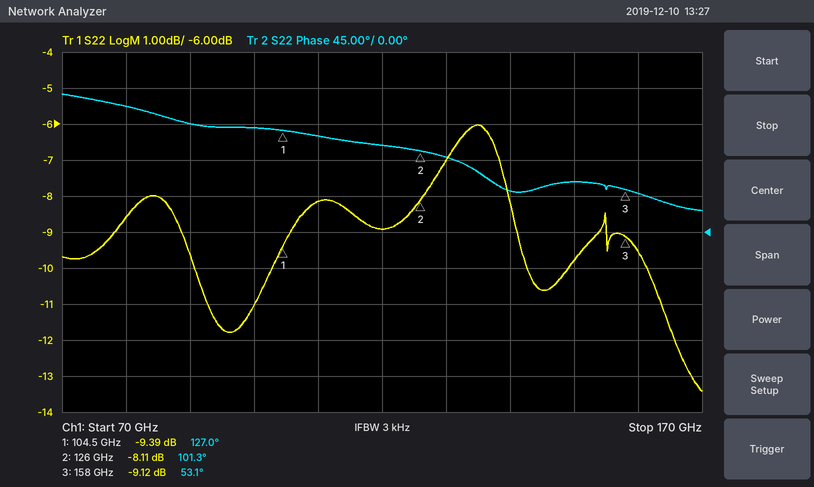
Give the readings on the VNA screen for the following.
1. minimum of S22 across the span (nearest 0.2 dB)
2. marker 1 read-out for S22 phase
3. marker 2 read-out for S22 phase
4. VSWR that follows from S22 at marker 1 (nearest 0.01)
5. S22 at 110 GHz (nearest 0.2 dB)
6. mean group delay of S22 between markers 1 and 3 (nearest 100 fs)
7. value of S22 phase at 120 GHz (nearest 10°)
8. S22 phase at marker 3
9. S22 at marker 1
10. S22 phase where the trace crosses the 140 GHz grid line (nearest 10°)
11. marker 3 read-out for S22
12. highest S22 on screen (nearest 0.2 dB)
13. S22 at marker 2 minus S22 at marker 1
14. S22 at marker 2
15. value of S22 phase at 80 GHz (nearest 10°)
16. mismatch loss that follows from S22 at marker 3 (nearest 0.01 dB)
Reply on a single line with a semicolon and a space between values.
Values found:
-13.4 dB; 127.0°; 101.3°; 2.03; -8.2 dB; 3.8 ps; 110°; 53.1°; -9.39 dB; 50°; -9.12 dB; -6.0 dB; 1.28 dB; -8.11 dB; 160°; 0.57 dB
